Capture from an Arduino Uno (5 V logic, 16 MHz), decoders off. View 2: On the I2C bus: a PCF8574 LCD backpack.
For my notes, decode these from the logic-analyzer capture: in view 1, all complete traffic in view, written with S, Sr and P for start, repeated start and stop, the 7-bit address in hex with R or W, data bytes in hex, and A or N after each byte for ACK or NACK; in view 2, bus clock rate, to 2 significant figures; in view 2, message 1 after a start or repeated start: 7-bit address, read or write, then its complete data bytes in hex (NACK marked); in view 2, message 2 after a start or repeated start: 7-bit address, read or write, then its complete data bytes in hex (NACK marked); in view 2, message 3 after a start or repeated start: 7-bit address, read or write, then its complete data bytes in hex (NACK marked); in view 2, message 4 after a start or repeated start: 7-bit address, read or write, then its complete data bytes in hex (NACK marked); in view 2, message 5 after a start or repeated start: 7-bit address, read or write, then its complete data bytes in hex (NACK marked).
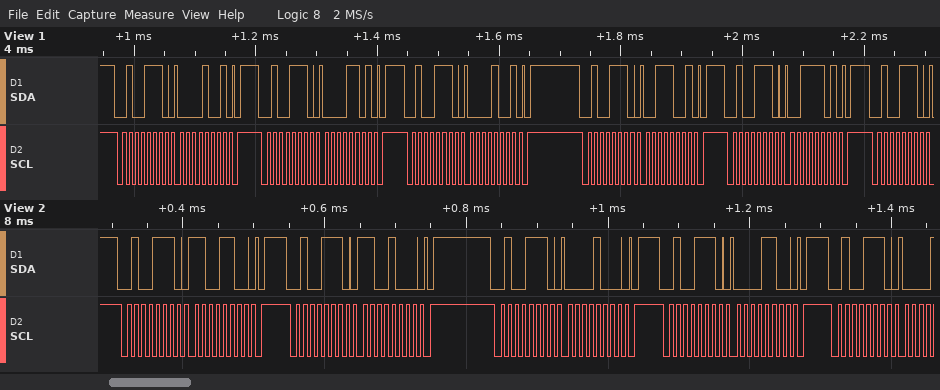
S 27W A 09 A P S 27W A 0D A P S 27W A 09 A P S 27W A 39 A P S 27W A 3D A P S 27W A
100 kHz
0x27 write: CC
0x27 write: C8
0x27 write: 08
0x27 write: 0C
0x27 write
